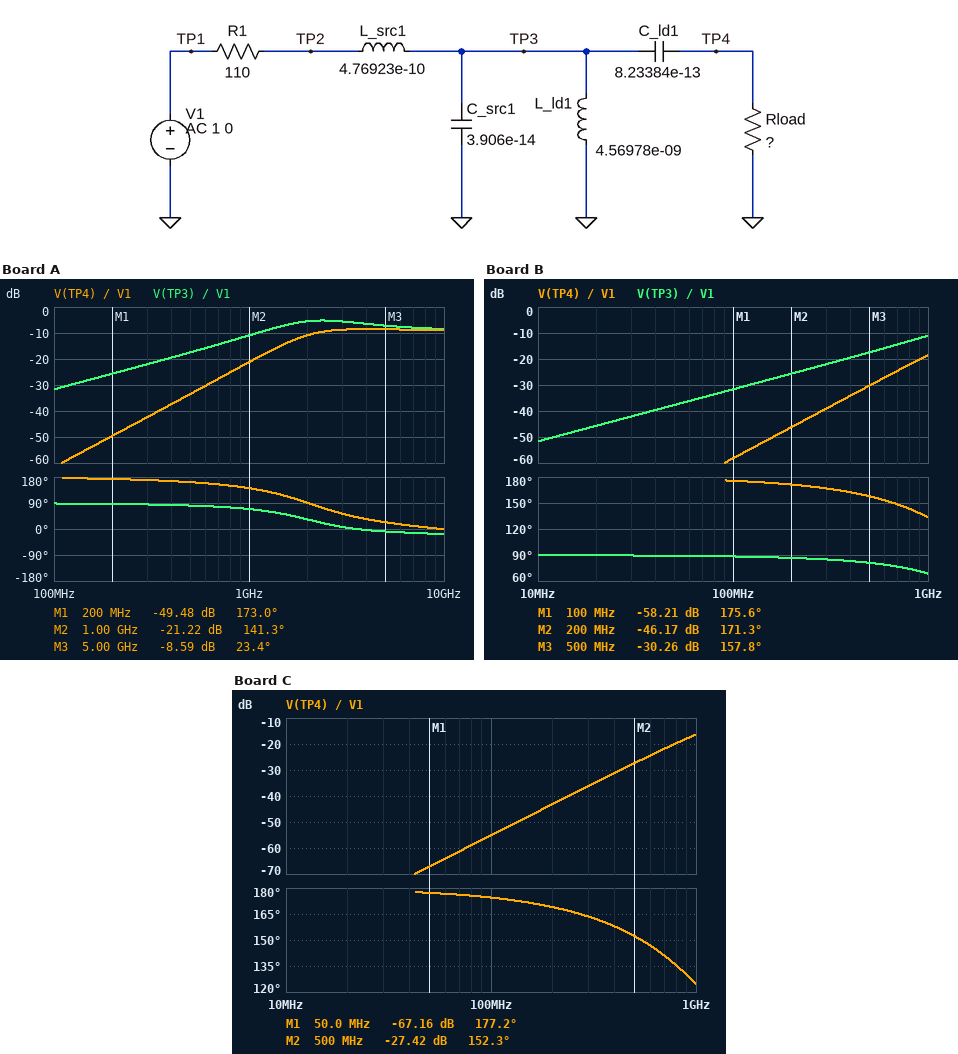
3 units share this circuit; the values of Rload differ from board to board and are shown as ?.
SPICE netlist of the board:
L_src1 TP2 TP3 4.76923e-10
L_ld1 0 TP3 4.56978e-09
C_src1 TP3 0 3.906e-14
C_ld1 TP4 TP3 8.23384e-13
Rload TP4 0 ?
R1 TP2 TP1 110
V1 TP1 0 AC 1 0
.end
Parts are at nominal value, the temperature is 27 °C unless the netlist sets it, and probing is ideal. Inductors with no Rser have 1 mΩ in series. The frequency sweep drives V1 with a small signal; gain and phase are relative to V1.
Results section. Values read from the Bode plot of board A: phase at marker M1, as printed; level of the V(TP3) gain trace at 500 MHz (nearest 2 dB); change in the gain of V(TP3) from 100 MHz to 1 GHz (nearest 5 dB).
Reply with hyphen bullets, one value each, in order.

- 173.0 deg
- -18 dB
- 20 dB
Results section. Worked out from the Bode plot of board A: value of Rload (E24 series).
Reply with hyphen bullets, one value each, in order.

- 62 Ω
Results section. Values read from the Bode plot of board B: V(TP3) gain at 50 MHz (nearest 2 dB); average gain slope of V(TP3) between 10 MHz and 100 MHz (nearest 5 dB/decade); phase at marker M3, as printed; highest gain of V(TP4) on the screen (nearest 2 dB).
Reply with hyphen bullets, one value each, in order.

- -38 dB
- 20 dB/decade
- 157.8 deg
- -18 dB
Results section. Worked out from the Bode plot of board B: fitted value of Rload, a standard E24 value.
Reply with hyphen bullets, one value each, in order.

- 91 Ω
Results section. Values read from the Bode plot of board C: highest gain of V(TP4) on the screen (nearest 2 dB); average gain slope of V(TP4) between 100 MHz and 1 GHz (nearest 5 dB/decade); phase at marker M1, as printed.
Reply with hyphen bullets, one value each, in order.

- -16 dB
- 40 dB/decade
- 177.2 deg
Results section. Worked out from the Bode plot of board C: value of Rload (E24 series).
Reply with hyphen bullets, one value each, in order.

- 130 Ω
